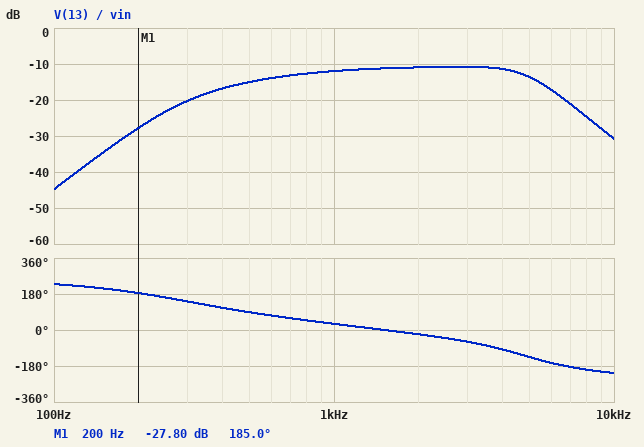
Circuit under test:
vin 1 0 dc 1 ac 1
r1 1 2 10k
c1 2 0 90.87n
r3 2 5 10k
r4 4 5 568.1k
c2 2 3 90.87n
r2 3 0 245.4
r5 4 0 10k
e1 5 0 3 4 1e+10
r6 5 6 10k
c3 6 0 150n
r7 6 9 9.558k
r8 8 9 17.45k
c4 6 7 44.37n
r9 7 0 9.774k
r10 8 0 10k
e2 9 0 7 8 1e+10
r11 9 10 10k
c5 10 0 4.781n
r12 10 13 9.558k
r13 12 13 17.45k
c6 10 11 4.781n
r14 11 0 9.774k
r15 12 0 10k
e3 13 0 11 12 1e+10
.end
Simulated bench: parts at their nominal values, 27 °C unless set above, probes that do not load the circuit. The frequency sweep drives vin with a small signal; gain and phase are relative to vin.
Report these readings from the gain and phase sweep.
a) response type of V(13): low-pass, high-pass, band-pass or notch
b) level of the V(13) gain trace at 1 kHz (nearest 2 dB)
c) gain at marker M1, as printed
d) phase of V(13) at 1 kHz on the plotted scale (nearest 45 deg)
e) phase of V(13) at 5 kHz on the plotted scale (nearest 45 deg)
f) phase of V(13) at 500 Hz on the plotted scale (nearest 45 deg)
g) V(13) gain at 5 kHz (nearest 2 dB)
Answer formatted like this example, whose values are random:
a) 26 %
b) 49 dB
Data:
a) band-pass
b) -12 dB
c) -27.80 dB
d) 45 deg
e) -135 deg
f) 90 deg
g) -14 dB
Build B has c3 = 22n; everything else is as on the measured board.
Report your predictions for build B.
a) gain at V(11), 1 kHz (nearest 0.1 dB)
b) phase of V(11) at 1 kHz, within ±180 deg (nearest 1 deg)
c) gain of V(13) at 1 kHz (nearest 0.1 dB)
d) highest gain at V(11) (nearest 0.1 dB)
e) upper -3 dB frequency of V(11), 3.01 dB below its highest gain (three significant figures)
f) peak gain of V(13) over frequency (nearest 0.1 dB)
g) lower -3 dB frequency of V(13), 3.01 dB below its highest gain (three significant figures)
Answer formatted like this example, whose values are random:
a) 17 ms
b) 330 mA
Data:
a) -0.8 dB
b) 56 deg
c) 8.0 dB
d) -0.7 dB
e) 4.26 kHz
f) 8.1 dB
g) 658 Hz
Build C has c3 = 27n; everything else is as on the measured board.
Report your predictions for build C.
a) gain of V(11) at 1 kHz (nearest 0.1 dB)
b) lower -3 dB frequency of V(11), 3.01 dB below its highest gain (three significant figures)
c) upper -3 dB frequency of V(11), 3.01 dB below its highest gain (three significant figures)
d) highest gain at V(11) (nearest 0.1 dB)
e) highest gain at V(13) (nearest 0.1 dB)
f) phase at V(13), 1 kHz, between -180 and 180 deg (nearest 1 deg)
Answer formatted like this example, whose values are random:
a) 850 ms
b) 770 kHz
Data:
a) -3.2 dB
b) 602 Hz
c) 4.52 kHz
d) -3.1 dB
e) 5.7 dB
f) 49 deg
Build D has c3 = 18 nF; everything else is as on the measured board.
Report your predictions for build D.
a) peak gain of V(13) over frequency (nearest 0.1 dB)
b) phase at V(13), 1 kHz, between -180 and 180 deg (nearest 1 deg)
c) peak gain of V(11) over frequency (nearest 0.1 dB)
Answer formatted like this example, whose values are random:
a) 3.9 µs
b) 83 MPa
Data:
a) 10.4 dB
b) 66 deg
c) 1.6 dB
